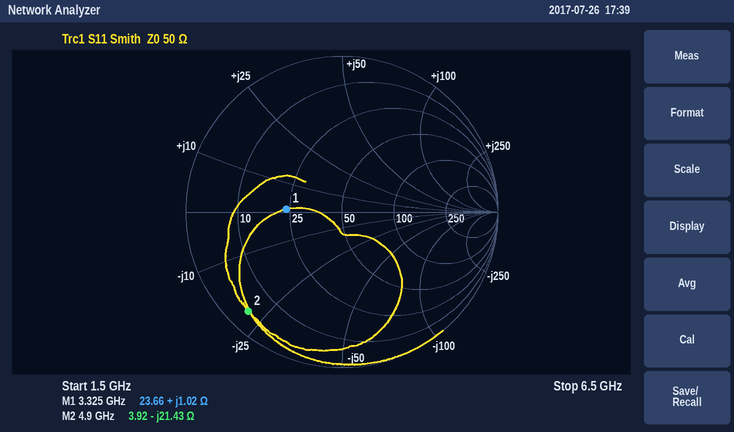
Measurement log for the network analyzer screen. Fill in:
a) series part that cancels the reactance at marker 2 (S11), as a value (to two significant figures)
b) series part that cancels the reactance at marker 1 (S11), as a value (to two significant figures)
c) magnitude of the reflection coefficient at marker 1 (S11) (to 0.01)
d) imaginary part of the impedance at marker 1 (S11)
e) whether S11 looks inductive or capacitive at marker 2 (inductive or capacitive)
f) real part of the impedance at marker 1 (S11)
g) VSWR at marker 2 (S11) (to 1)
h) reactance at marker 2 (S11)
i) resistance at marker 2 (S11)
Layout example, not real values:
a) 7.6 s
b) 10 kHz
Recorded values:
a) 700 pH
b) 47 pF
c) 0.36
d) +1.02 Ω
e) capacitive
f) 23.66 Ω
g) 15
h) -21.43 Ω
i) 3.92 Ω
